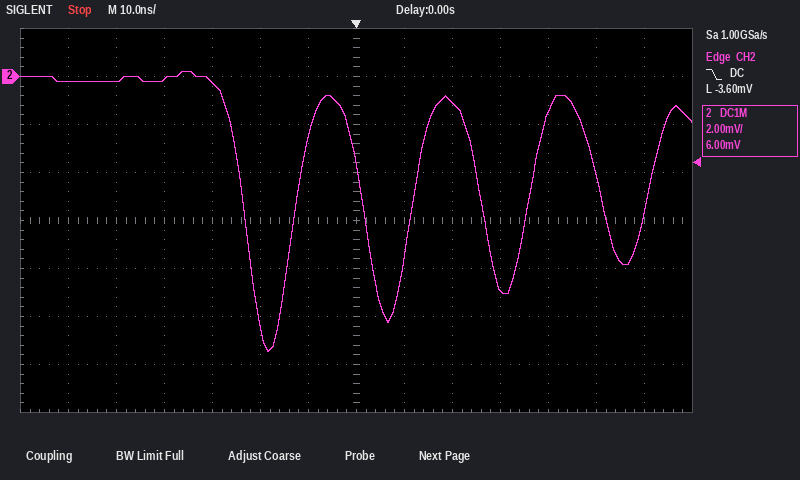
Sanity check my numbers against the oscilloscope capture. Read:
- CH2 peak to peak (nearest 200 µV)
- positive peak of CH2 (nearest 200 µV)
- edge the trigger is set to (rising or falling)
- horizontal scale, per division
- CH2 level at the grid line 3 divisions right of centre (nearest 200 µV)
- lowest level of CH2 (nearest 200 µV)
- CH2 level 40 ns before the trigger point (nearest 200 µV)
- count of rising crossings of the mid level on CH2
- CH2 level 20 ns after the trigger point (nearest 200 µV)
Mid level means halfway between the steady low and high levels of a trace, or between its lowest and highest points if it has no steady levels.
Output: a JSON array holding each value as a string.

["11.6 mV", "200 µV", "falling", "10 ns", "-8.8 mV", "-11.4 mV", "-200 µV", "4", "-1.0 mV"]
